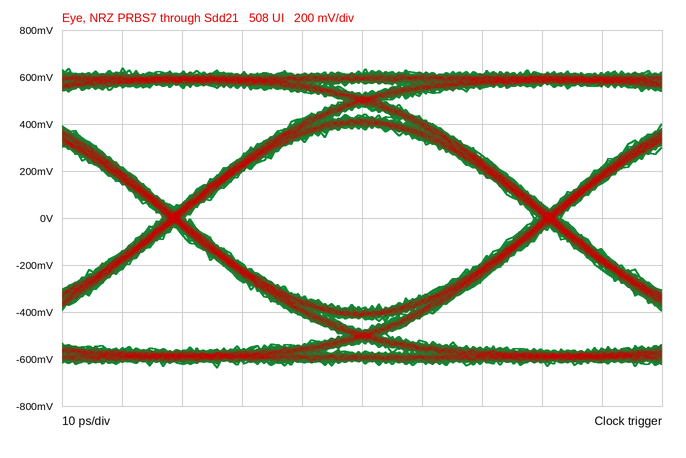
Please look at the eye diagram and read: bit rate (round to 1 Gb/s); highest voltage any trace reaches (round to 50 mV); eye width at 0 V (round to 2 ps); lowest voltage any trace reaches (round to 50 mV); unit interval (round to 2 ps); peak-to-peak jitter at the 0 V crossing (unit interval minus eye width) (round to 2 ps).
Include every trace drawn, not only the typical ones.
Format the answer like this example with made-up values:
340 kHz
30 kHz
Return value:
16 Gb/s
650 mV
58 ps
-650 mV
62 ps
4 ps
